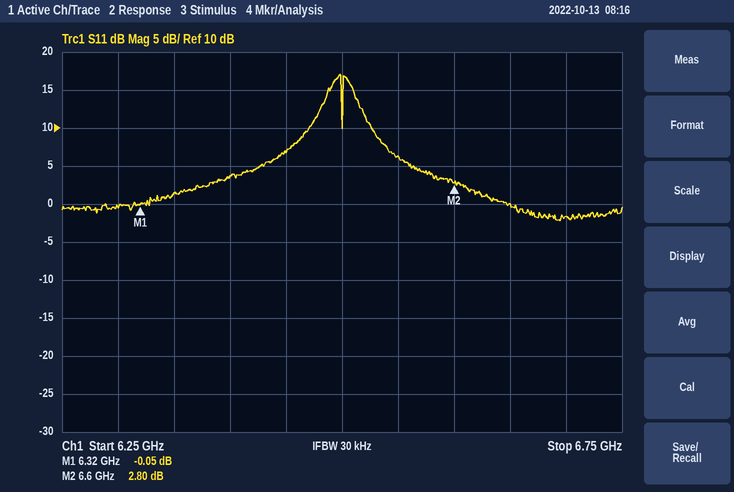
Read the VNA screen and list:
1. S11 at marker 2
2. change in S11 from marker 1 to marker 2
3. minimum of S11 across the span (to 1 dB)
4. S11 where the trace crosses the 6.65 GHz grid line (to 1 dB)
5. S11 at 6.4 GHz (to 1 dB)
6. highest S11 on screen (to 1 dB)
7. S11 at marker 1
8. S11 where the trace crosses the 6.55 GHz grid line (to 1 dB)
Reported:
2.80 dB
2.85 dB
-2 dB
0 dB
4 dB
17 dB
-0.05 dB
6 dB
